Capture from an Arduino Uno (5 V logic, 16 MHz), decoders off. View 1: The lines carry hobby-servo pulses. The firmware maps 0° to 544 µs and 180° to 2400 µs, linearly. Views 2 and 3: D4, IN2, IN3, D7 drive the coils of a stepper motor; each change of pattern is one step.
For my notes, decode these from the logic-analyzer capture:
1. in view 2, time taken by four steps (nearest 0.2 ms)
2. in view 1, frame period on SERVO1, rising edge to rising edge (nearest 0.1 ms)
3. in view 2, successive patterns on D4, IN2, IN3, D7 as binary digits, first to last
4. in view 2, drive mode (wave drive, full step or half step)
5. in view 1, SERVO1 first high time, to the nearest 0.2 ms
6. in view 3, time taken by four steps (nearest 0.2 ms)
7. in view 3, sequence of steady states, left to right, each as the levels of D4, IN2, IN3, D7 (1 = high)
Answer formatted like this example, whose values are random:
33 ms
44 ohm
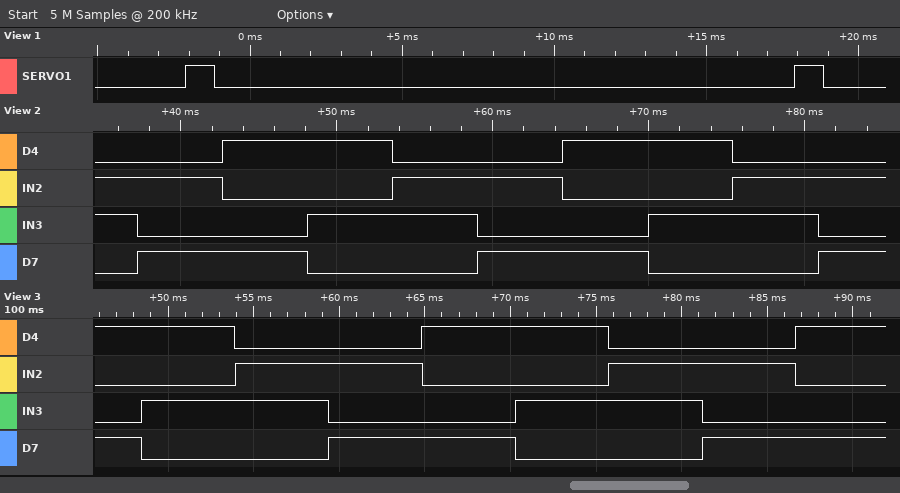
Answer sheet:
21.8 ms
20.0 ms
0110 0101 1001 1010 0110 0101 1001 1010 0110 0101
full step
1.0 ms
21.8 ms
1001 1010 0110 0101 1001 1010 0110 0101 1001
